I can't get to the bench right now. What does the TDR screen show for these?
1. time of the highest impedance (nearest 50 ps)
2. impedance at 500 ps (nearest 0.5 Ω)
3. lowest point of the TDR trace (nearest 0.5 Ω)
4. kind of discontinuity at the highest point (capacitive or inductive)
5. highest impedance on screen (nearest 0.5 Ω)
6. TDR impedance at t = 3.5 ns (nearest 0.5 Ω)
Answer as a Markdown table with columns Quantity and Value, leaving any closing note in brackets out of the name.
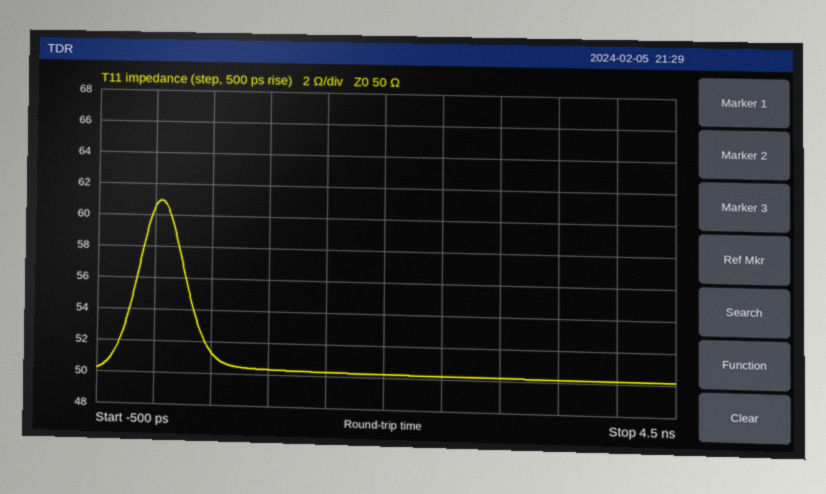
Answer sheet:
| Quantity | Value |
|---|---|
| time of the highest impedance | 50 ps |
| impedance at 500 ps | 51.5 Ω |
| lowest point of the TDR trace | 50.0 Ω |
| kind of discontinuity at the highest point | inductive |
| highest impedance on screen | 61.0 Ω |
| TDR impedance at t = 3.5 ns | 50.0 Ω |
